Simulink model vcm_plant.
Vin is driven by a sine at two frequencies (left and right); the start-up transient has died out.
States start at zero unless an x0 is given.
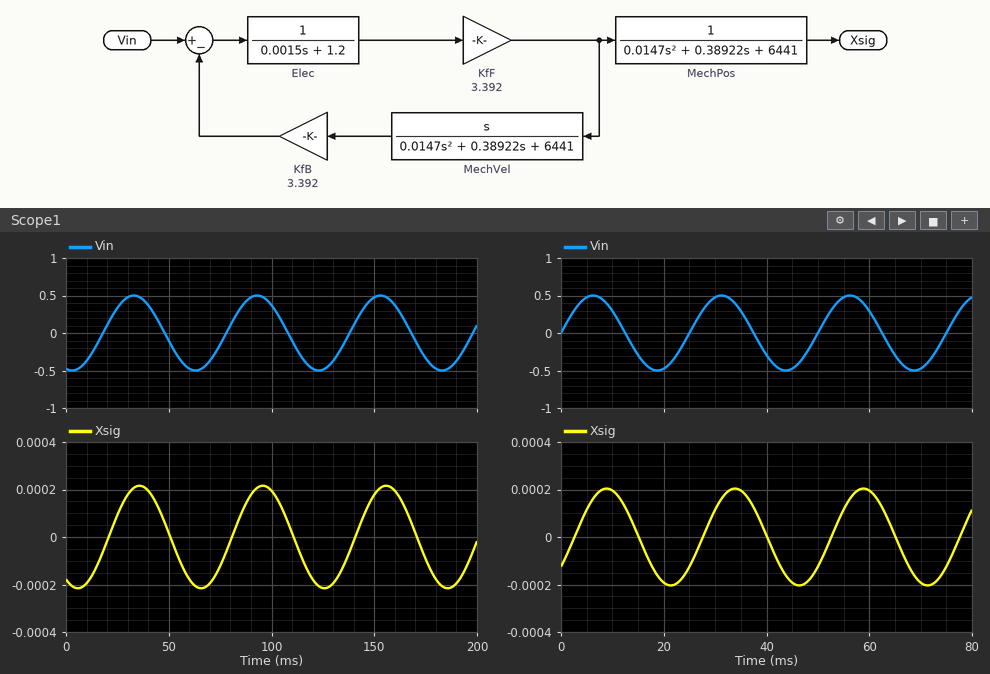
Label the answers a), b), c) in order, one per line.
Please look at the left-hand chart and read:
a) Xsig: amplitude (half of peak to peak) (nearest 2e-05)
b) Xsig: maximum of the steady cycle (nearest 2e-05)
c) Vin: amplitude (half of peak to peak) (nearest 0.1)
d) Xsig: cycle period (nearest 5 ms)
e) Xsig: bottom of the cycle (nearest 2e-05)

a) 0.00022
b) 0.00022
c) 0.5
d) 60 ms
e) -0.00022
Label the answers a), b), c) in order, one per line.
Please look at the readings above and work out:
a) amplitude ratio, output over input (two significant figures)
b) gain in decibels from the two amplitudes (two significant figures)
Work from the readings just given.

a) 0.00044
b) -67 dB
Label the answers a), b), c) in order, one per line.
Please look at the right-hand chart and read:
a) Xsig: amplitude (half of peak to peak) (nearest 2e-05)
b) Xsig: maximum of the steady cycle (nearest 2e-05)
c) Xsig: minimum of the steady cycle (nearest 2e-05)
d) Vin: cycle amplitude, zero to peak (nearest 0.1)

a) 0.00020
b) 0.00020
c) -0.00020
d) 0.5
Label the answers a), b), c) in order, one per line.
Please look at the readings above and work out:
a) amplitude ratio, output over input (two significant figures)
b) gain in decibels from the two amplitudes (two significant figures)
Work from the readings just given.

a) 0.00040
b) -68 dB
